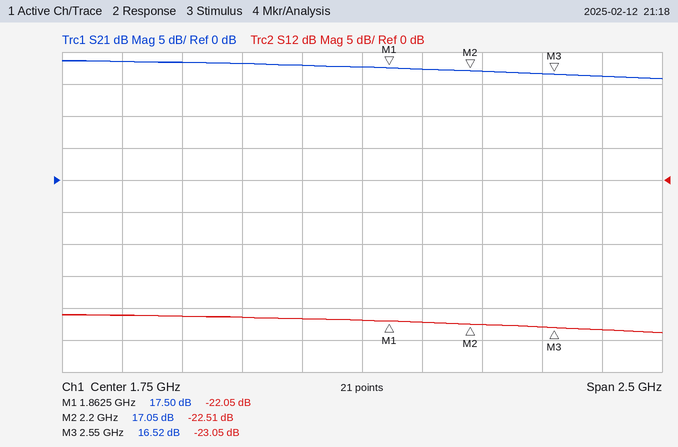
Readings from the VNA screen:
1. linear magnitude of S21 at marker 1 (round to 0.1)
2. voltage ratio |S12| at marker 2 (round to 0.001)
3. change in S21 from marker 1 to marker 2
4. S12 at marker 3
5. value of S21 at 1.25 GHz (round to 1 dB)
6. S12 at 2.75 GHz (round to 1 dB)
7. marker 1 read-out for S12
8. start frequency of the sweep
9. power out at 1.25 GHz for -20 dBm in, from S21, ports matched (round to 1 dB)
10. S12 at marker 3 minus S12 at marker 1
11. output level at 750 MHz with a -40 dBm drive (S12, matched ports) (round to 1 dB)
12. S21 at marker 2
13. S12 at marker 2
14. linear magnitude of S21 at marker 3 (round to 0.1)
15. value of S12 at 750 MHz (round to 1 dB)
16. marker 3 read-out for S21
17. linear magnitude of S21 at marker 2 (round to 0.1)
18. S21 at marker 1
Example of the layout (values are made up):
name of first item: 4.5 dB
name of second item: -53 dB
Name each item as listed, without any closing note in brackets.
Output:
linear magnitude of S21 at marker 1: 7.5
voltage ratio |S12| at marker 2: 0.075
change in S21 from marker 1 to marker 2: -0.45 dB
S12 at marker 3: -23.05 dB
value of S21 at 1.25 GHz: 18 dB
S12 at 2.75 GHz: -23 dB
marker 1 read-out for S12: -22.05 dB
start frequency of the sweep: 500 MHz
power out at 1.25 GHz for -20 dBm in, from S21, ports matched: -2 dBm
S12 at marker 3 minus S12 at marker 1: -1.00 dB
output level at 750 MHz with a -40 dBm drive (S12, matched ports): -61 dBm
S21 at marker 2: 17.05 dB
S12 at marker 2: -22.51 dB
linear magnitude of S21 at marker 3: 6.7
value of S12 at 750 MHz: -21 dB
marker 3 read-out for S21: 16.52 dB
linear magnitude of S21 at marker 2: 7.1
S21 at marker 1: 17.50 dB
